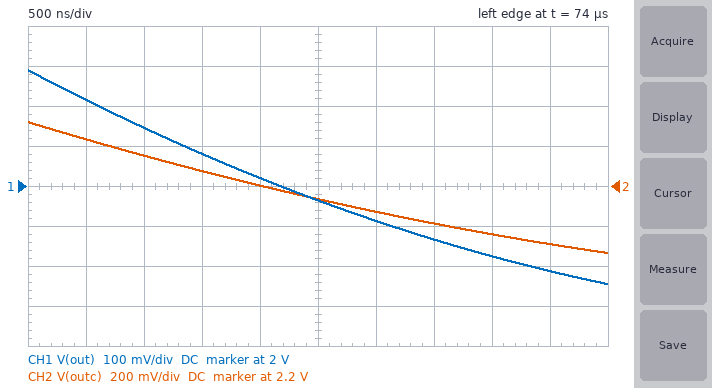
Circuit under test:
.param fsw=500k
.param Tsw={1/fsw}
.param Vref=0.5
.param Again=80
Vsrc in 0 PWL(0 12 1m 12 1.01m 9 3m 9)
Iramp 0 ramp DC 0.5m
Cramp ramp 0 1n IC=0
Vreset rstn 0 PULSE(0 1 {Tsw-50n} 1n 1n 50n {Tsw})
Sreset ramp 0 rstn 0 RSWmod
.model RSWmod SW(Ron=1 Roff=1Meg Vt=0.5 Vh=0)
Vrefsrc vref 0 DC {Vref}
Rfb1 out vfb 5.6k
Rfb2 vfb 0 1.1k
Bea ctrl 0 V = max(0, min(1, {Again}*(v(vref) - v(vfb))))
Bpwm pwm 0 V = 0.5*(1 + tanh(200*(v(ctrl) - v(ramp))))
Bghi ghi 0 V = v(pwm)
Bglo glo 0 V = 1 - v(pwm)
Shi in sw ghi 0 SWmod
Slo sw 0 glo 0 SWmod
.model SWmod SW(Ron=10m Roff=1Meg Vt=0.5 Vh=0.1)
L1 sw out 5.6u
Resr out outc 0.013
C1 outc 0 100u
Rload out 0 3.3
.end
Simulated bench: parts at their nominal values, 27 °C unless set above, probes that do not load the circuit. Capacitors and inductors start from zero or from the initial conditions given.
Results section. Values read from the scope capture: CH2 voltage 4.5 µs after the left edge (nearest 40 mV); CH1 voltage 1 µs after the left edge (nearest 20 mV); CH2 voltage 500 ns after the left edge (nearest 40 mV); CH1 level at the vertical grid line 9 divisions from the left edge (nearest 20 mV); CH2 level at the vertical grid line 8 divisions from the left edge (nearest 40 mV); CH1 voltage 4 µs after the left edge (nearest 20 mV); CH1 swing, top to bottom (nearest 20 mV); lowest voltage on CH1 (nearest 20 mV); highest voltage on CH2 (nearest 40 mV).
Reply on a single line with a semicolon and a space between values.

1.92 V; 2.14 V; 2.44 V; 1.78 V; 1.96 V; 1.82 V; 540 mV; 1.76 V; 2.52 V
